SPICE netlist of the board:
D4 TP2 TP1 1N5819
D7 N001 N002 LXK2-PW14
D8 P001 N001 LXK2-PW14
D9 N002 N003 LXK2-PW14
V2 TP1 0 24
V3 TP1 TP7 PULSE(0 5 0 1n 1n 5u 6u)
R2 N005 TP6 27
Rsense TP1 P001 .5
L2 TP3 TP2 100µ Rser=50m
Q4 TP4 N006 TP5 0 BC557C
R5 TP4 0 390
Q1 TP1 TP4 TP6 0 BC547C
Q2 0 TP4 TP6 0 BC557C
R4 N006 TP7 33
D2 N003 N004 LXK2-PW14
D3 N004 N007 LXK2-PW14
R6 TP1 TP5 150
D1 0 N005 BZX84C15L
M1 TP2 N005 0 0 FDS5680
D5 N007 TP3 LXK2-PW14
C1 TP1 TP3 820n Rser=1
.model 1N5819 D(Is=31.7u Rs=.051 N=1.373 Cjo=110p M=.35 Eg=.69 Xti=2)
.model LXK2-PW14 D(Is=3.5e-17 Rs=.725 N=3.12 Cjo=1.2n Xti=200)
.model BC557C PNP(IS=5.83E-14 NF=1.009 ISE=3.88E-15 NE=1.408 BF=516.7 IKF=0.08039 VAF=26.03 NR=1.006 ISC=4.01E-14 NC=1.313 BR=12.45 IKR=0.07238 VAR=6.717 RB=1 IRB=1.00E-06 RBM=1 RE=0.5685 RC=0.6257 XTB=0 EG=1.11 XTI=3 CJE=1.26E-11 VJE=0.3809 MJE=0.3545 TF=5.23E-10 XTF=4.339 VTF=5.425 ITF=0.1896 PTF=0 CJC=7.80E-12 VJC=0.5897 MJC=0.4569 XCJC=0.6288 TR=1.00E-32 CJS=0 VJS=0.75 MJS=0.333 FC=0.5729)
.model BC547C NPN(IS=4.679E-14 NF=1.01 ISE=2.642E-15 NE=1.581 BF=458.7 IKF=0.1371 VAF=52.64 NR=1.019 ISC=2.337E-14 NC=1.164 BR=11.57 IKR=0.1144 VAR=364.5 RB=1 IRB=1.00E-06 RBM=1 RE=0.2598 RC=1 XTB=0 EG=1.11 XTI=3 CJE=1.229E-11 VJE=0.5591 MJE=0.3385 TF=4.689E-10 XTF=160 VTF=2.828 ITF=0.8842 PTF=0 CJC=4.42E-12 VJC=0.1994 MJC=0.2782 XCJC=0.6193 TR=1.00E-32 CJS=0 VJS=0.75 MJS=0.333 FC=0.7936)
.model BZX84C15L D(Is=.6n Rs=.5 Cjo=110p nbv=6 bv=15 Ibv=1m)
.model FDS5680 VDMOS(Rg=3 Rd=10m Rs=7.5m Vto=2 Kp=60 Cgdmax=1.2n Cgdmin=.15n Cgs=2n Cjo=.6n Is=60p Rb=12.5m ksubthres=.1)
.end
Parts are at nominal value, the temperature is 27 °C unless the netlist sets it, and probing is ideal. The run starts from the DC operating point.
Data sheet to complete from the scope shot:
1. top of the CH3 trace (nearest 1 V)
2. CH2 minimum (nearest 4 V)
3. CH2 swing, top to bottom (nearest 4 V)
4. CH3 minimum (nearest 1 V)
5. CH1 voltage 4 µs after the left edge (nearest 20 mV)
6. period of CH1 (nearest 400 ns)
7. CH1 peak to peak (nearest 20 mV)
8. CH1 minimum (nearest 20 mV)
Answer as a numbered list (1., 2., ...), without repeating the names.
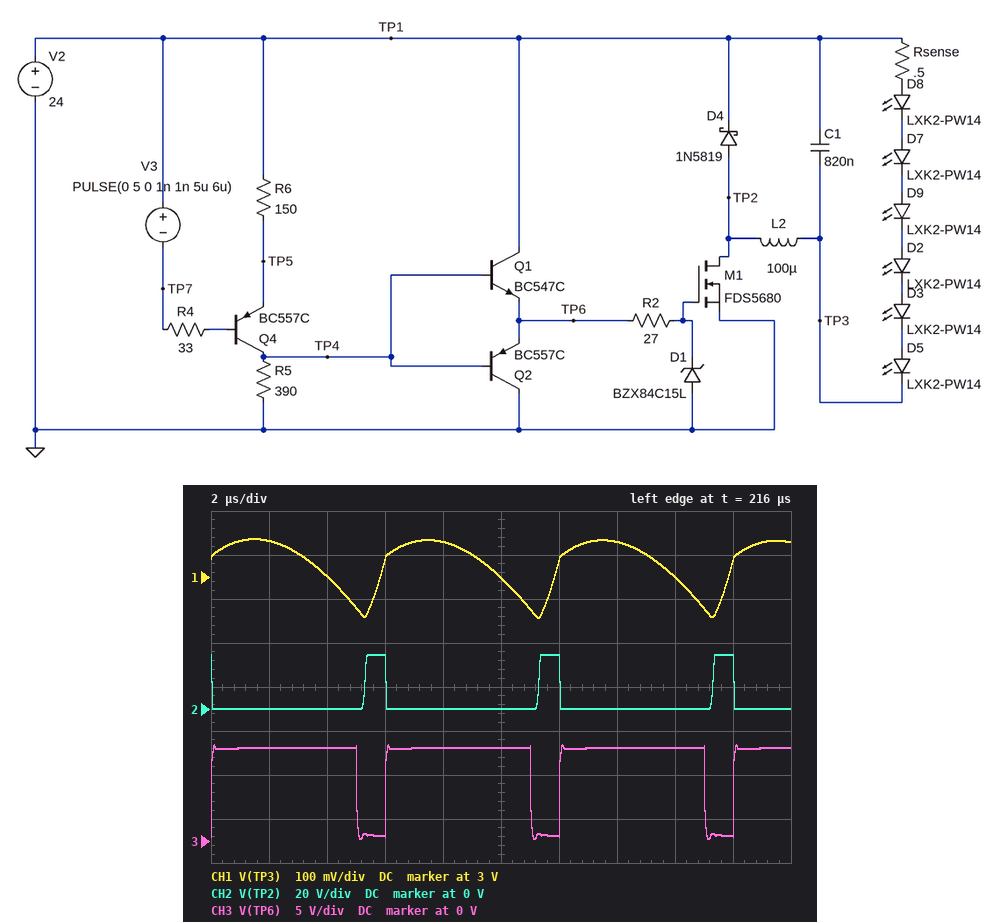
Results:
1. 11 V
2. 0 V
3. 24 V
4. 0 V
5. 3.00 V
6. 6.0 µs
7. 180 mV
8. 2.90 V
